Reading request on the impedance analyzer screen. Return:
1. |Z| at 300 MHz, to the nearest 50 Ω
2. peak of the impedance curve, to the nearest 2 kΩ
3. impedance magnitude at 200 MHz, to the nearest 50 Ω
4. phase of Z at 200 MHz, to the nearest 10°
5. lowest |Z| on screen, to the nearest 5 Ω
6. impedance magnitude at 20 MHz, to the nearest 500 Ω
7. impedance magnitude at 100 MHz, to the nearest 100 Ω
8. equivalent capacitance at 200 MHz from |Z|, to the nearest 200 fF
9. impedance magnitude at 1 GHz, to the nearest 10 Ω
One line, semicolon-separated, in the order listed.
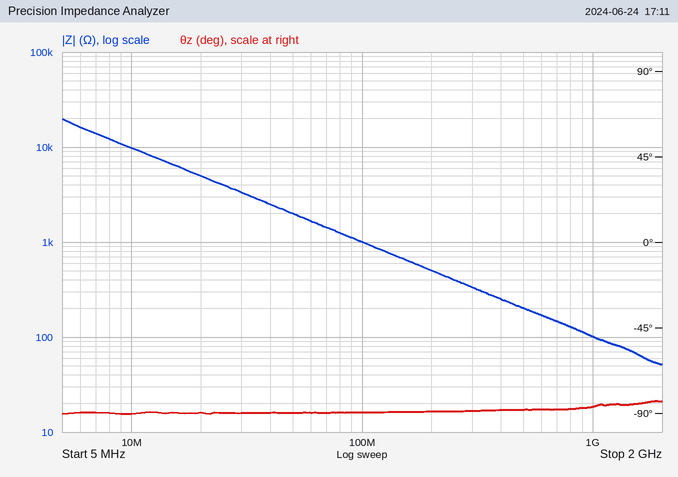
350 Ω; 20 kΩ; 500 Ω; -90°; 50 Ω; 5.0 kΩ; 1.0 kΩ; 1.6 pF; 100 Ω
